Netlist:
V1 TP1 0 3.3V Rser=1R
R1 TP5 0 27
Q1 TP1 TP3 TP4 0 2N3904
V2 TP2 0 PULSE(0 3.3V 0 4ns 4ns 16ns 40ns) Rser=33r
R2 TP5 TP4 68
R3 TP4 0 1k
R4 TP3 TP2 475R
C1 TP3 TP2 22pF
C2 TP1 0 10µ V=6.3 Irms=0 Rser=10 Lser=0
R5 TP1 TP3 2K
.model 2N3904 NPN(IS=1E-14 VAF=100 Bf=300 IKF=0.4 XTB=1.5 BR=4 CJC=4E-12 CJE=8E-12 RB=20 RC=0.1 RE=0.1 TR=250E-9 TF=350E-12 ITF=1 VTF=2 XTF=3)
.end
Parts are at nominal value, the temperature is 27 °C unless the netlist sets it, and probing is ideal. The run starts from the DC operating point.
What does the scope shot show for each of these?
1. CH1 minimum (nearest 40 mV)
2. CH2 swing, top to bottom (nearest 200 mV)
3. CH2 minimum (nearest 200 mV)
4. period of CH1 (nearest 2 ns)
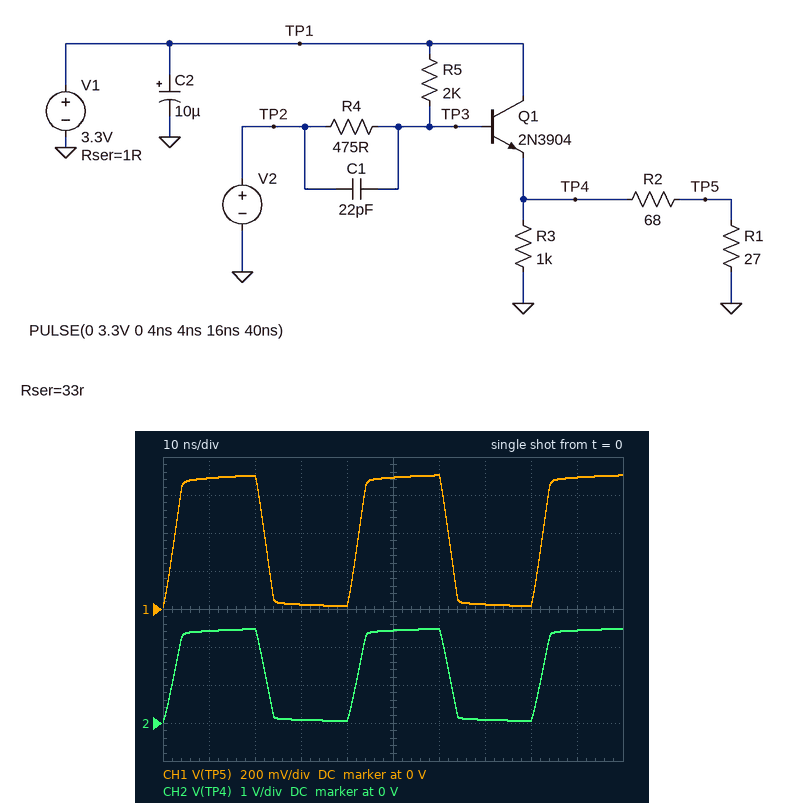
0 V
2.4 V
0 V
40 ns
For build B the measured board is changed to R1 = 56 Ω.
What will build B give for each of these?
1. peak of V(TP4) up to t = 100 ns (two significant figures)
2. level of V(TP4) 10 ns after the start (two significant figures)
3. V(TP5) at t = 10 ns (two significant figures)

2.5 V
2.5 V
1.1 V
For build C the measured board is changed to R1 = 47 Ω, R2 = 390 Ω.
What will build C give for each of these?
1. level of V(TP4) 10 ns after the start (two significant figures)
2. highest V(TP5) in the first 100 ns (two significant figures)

2.6 V
280 mV
